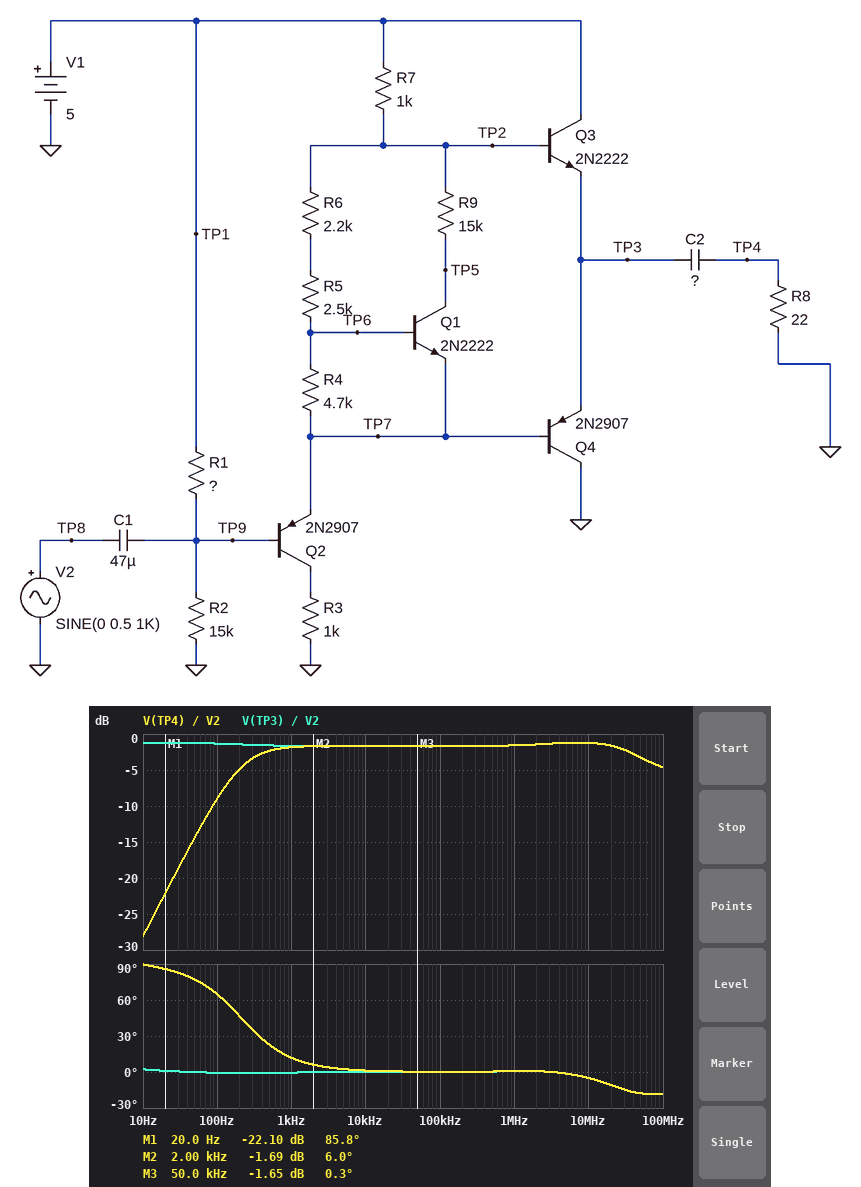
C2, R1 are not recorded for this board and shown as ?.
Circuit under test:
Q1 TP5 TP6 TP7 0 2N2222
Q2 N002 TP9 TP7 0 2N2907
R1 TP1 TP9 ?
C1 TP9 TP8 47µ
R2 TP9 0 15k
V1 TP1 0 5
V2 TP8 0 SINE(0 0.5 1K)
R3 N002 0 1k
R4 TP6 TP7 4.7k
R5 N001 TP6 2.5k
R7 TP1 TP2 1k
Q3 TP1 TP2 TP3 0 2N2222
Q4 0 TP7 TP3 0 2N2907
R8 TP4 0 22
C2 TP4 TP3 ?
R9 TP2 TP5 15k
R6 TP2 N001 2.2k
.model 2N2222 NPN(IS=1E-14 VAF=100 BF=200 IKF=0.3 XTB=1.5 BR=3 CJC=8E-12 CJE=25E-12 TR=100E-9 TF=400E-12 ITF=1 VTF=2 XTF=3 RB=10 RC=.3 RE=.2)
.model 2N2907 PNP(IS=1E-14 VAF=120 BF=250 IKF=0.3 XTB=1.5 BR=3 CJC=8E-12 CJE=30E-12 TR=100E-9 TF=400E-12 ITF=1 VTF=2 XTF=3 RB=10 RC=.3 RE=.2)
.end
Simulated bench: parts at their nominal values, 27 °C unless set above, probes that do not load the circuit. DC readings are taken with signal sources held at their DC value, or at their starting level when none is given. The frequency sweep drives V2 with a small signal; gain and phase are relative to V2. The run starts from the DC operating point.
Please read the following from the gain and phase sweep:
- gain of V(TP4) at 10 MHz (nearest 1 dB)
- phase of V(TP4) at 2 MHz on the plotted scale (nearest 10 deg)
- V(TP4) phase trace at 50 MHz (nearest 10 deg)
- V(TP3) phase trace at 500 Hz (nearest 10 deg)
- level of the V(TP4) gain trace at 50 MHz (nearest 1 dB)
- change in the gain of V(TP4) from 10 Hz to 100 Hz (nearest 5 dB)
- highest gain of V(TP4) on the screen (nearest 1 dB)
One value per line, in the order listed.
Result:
-1 dB
0 deg
-20 deg
0 deg
-3 dB
20 dB
-1 dB
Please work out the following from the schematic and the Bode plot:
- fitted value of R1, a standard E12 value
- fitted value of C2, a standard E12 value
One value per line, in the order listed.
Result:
18 kΩ
33 µF
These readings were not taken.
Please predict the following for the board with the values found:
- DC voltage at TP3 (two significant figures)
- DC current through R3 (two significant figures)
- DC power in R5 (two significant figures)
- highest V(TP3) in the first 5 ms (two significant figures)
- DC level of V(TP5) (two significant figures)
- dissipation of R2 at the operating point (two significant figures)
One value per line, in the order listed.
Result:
3.7 V
490 µA
93 µW
4.0 V
2.9 V
350 µW
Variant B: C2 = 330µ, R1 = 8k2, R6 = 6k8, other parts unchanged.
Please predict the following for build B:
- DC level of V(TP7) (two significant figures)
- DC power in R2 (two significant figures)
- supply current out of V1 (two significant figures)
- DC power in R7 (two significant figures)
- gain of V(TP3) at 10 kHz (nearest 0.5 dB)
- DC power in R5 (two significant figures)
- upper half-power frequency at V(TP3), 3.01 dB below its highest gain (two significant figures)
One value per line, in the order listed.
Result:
3.8 V
700 µW
310 µA
6.2 µW
-36.5 dB
15 µW
1.8 GHz
